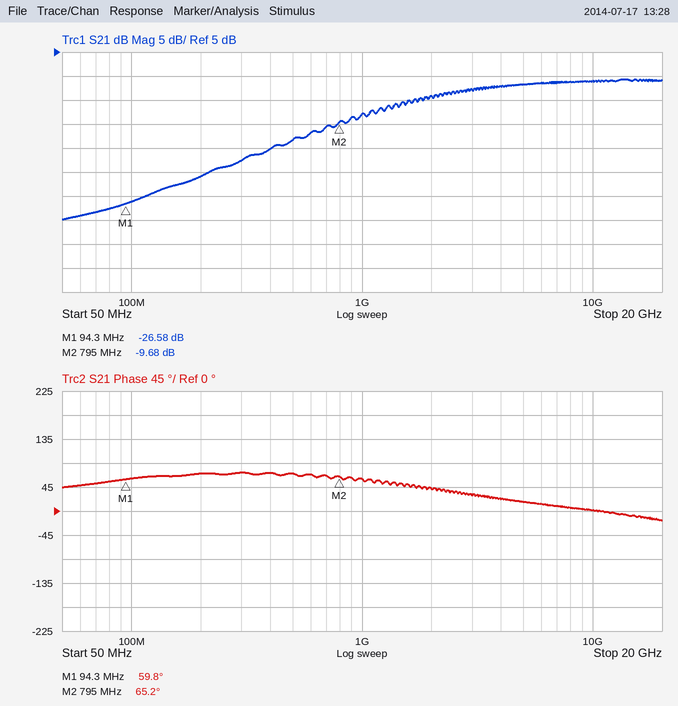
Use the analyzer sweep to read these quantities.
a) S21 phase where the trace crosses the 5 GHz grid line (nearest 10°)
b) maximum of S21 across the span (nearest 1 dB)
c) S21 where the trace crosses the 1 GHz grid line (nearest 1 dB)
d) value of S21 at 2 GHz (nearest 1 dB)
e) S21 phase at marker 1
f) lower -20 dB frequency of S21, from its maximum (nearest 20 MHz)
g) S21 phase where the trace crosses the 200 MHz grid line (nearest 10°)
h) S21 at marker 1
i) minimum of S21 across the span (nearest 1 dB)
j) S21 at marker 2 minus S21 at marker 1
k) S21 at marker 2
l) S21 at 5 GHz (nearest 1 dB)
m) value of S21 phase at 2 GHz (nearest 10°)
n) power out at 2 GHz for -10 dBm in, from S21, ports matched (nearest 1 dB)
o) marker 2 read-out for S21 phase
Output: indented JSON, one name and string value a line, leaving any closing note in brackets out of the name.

{
  "S21 phase where the trace crosses the 5 GHz grid line": "20°",
  "maximum of S21 across the span": "-1 dB",
  "S21 where the trace crosses the 1 GHz grid line": "-8 dB",
  "value of S21 at 2 GHz": "-4 dB",
  "S21 phase at marker 1": "59.8°",
  "lower -20 dB frequency of S21, from its maximum": "200 MHz",
  "S21 phase where the trace crosses the 200 MHz grid line": "70°",
  "S21 at marker 1": "-26.58 dB",
  "minimum of S21 across the span": "-30 dB",
  "S21 at marker 2 minus S21 at marker 1": "16.90 dB",
  "S21 at marker 2": "-9.68 dB",
  "S21 at 5 GHz": "-2 dB",
  "value of S21 phase at 2 GHz": "40°",
  "power out at 2 GHz for -10 dBm in, from S21, ports matched": "-14 dBm",
  "marker 2 read-out for S21 phase": "65.2°"
}
